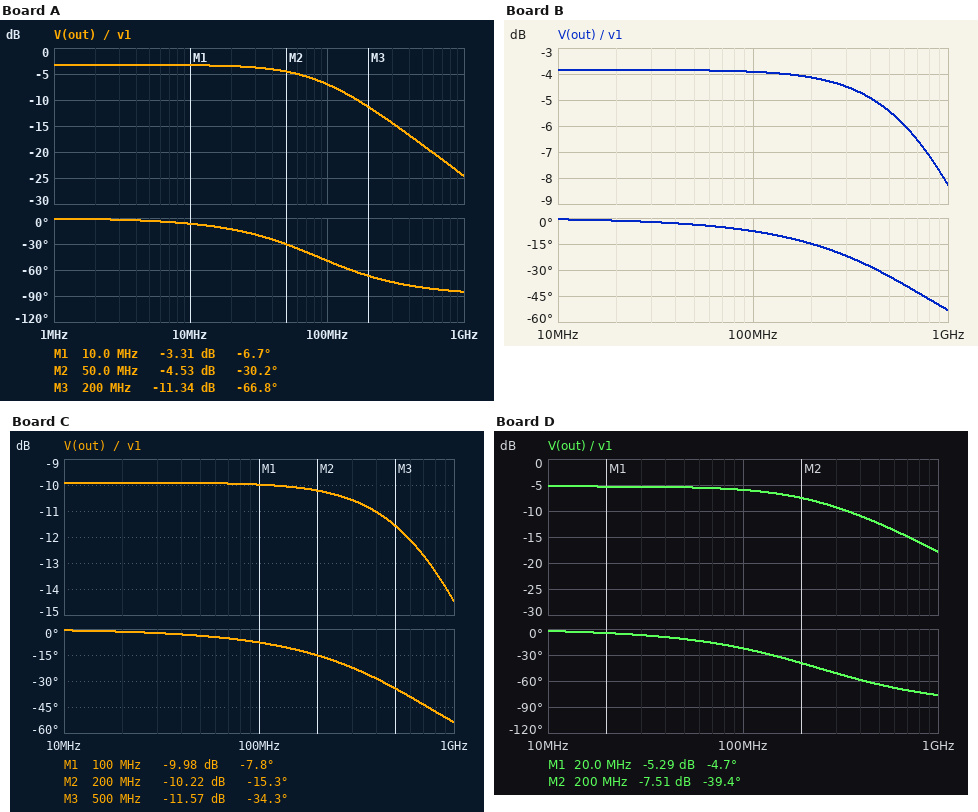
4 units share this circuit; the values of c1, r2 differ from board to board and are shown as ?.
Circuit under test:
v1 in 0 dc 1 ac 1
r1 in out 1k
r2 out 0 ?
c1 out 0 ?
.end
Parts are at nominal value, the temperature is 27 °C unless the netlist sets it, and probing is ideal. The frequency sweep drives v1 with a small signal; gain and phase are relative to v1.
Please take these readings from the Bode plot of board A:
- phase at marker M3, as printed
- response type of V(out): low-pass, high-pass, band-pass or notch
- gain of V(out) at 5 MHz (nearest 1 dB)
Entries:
-66.8 deg
low-pass
-3 dB
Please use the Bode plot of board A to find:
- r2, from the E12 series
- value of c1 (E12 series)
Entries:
2.2 kΩ
2.7 pF
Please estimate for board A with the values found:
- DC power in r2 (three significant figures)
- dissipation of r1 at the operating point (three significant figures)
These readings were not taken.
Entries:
215 µW
97.7 µW
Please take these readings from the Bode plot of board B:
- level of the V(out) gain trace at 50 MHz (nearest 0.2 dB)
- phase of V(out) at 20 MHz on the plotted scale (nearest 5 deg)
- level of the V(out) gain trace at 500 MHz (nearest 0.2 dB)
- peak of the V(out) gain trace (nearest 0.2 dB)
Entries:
-3.8 dB
0 deg
-5.4 dB
-3.8 dB
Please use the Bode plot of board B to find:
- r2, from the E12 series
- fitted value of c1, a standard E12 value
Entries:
1.8 kΩ
330 fF
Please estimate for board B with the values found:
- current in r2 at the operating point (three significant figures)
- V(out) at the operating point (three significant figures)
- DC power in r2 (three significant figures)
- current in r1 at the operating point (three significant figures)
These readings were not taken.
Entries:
357 µA
643 mV
230 µW
357 µA
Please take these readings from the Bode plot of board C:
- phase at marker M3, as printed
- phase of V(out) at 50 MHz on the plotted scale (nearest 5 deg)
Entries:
-34.3 deg
-5 deg
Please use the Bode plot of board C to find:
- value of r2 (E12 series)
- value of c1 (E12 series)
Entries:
470 Ω
680 fF
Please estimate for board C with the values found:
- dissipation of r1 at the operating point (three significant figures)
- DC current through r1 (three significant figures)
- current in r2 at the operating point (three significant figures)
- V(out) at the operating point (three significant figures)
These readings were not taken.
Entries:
463 µW
680 µA
680 µA
320 mV
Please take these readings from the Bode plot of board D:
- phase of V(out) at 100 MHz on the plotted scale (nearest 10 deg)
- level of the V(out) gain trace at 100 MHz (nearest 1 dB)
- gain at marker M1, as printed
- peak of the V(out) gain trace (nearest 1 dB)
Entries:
-20 deg
-6 dB
-5.29 dB
-5 dB
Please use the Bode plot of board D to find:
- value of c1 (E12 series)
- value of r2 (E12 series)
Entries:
1.2 pF
1.2 kΩ
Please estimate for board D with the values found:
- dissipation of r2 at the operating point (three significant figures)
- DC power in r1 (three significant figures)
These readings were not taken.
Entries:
248 µW
207 µW
